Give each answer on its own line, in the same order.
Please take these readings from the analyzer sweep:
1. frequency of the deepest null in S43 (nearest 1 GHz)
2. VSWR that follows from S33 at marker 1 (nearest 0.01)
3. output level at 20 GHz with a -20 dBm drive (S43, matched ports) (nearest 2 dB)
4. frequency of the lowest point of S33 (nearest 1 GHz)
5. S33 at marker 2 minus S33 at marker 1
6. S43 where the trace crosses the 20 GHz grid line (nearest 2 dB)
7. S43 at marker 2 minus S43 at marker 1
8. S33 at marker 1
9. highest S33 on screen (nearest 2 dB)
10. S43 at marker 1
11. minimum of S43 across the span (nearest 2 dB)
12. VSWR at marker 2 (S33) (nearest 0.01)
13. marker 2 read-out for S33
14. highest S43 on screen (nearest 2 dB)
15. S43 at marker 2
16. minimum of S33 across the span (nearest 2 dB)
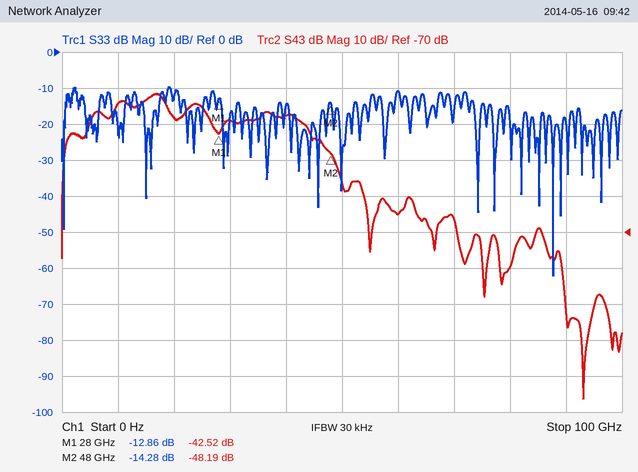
93 GHz
1.59
-58 dBm
88 GHz
-1.42 dB
-38 dB
-5.67 dB
-12.86 dB
-10 dB
-42.52 dB
-116 dB
1.48
-14.28 dB
-32 dB
-48.19 dB
-62 dB
